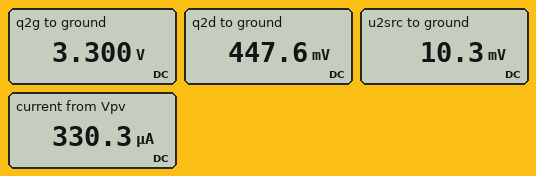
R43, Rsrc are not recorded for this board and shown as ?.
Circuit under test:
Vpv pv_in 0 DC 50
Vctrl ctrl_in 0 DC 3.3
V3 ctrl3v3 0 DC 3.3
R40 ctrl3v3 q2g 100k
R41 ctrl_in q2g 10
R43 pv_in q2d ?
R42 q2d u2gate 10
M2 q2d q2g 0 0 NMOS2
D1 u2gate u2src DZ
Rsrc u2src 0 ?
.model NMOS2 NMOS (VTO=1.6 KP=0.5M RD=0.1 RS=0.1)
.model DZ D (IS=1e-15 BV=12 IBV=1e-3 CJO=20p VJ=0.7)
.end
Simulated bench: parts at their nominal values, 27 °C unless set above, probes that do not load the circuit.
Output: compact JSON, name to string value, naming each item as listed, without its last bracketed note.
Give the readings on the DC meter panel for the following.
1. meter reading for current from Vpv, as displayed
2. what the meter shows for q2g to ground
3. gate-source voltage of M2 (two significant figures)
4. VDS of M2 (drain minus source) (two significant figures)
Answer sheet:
{"meter reading for current from Vpv, as displayed": "330.3 µA", "what the meter shows for q2g to ground": "3.300 V", "gate-source voltage of M2": "3.3 V", "VDS of M2 (drain minus source)": "450 mV"}
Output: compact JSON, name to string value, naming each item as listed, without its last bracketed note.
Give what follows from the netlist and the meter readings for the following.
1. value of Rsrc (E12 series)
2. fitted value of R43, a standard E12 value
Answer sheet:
{"value of Rsrc": "470 kΩ", "fitted value of R43, a standard E12 value": "150 kΩ"}
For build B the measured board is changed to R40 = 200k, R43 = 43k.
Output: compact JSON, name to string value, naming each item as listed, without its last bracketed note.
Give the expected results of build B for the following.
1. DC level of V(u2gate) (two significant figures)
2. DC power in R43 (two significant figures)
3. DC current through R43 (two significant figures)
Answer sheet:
{"DC level of V(u2gate)": "17 V", "DC power in R43": "25 mW", "DC current through R43": "760 µA"}
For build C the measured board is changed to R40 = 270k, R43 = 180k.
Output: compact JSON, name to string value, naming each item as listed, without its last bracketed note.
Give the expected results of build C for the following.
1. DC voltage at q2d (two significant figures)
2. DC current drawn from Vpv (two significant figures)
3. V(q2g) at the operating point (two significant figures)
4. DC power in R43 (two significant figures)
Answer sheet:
{"DC voltage at q2d": "360 mV", "DC current drawn from Vpv": "280 µA", "V(q2g) at the operating point": "3.3 V", "DC power in R43": "14 mW"}
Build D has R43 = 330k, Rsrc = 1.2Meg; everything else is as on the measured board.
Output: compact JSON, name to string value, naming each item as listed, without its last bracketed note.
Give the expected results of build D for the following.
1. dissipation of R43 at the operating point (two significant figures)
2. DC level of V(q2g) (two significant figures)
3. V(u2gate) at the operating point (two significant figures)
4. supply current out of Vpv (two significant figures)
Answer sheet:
{"dissipation of R43 at the operating point": "7.5 mW", "DC level of V(q2g)": "3.3 V", "V(u2gate) at the operating point": "190 mV", "supply current out of Vpv": "150 µA"}
